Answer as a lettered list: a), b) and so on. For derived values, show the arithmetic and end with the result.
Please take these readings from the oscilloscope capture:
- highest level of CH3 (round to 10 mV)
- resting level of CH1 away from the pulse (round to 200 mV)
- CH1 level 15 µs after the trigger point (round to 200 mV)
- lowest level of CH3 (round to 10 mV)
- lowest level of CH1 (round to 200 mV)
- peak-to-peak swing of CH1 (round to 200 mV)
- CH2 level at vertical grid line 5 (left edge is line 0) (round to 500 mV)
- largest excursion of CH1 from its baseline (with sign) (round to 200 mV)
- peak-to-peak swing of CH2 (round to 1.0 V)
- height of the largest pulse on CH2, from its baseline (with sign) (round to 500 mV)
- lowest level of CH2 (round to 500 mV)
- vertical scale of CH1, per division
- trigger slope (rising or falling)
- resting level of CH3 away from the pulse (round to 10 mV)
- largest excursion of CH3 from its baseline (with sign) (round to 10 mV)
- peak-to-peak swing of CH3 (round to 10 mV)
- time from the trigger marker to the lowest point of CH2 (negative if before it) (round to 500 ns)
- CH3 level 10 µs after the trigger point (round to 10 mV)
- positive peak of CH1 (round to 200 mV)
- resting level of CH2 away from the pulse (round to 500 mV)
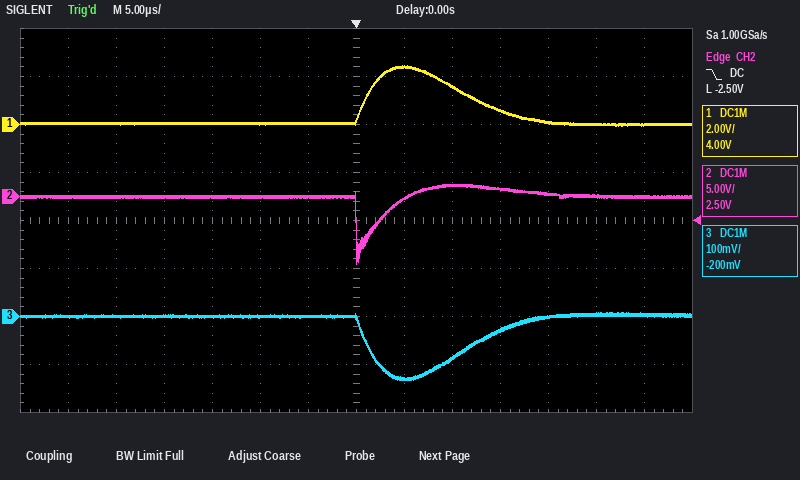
a) 10 mV
b) 0.0 V
c) 600 mV
d) -130 mV
e) 0.0 V
f) 2.4 V − (0.0 V) = 2.4 V
g) 0.0 V
h) 2.4 V − (0.0 V) = +2.4 V
i) 8.0 V
j) -7.0 V − (0.0 V) = -7.0 V
k) -7.0 V
l) 2 V
m) falling
n) 0 mV
o) -130 mV − (0 mV) = -130 mV
p) 10 mV − (-130 mV) = 140 mV
q) 0.0 µs
r) -90 mV
s) 2.4 V
t) 0.0 V
